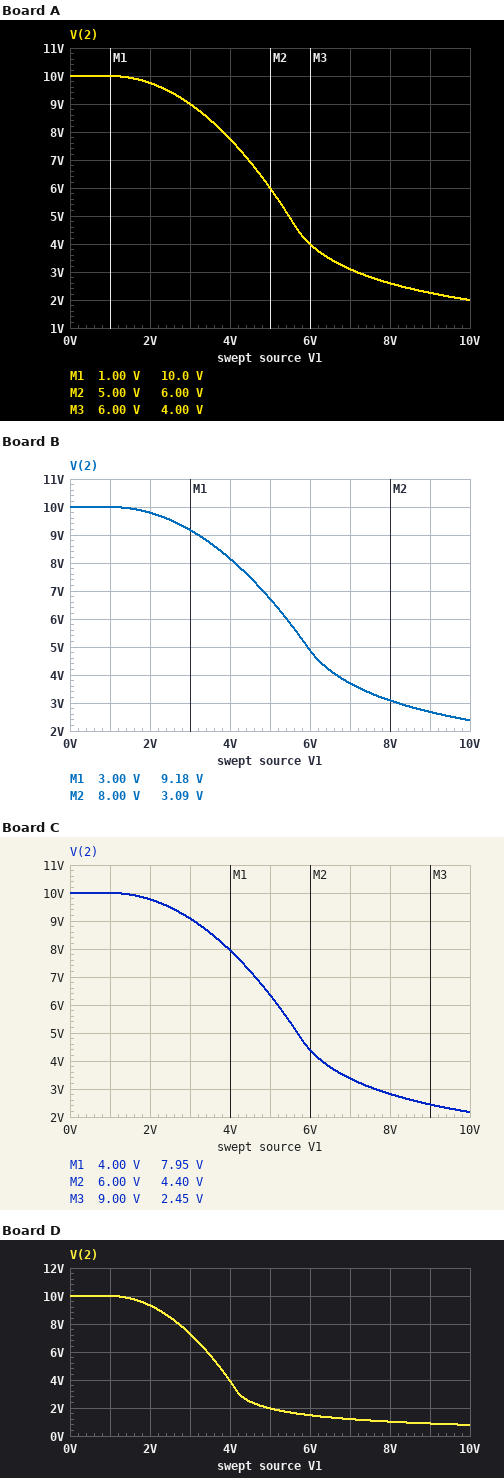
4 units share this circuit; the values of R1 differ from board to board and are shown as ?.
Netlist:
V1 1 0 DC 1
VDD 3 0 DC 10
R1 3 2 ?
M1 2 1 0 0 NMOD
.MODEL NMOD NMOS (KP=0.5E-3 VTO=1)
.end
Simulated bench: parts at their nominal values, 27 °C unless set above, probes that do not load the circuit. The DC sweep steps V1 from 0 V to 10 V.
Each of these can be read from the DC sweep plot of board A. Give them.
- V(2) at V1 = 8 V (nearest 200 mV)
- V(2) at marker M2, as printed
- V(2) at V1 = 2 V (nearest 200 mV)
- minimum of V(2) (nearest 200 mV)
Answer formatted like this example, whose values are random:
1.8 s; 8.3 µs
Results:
2.6 V; 6.00 V; 9.8 V; 2.0 V
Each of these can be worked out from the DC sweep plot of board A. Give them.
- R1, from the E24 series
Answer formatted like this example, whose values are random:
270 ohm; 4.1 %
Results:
1 kΩ
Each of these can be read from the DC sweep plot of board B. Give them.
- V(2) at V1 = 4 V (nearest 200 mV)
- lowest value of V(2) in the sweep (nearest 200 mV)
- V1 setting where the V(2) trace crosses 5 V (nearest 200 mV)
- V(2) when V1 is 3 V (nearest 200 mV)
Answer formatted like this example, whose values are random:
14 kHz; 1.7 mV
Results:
8.2 V; 2.4 V; 6.0 V; 9.2 V
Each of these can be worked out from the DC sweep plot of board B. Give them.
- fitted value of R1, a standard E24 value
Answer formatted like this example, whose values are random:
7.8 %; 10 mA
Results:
820 Ω
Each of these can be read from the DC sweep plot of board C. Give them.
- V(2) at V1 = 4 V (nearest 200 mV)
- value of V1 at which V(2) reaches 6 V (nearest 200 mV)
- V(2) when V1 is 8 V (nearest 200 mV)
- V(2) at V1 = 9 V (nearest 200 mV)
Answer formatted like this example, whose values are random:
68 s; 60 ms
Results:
8.0 V; 5.2 V; 2.8 V; 2.4 V
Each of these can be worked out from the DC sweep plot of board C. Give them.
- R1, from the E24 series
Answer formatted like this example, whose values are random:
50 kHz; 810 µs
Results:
910 Ω
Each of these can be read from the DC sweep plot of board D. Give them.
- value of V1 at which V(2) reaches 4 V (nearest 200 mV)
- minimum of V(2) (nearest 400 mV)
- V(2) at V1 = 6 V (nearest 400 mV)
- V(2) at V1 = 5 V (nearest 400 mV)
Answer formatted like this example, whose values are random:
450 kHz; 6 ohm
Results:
4.0 V; 800 mV; 1.6 V; 2.0 V
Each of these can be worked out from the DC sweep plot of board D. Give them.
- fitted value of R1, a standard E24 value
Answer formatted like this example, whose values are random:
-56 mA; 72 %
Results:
2.7 kΩ
